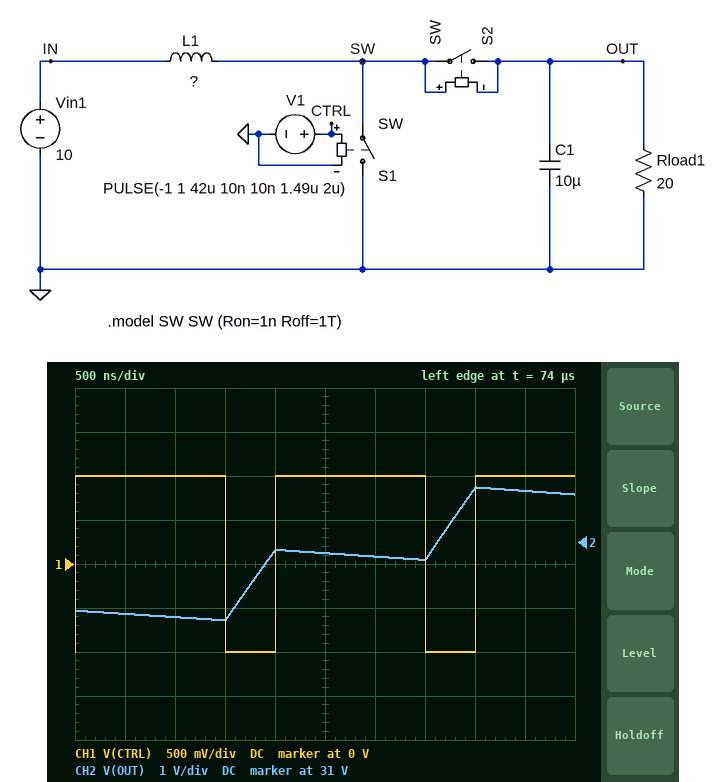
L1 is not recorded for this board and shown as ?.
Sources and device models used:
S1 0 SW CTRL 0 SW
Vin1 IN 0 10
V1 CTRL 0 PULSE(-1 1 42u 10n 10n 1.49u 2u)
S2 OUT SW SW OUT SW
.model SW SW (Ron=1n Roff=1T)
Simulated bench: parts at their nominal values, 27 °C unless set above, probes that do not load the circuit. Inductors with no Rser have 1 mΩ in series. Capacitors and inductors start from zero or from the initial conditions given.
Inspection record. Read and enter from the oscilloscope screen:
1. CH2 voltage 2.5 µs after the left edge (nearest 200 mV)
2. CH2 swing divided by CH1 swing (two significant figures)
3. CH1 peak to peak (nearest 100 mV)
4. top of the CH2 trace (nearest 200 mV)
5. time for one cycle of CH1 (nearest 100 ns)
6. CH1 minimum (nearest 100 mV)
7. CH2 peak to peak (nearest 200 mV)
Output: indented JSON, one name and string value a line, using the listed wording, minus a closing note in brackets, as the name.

{
  "CH2 voltage 2.5 µs after the left edge": "30.8 V",
  "CH2 swing divided by CH1 swing": "1.5",
  "CH1 peak to peak": "2.0 V",
  "top of the CH2 trace": "32.2 V",
  "time for one cycle of CH1": "2.0 µs",
  "CH1 minimum": "-1.0 V",
  "CH2 peak to peak": "3.0 V"
}
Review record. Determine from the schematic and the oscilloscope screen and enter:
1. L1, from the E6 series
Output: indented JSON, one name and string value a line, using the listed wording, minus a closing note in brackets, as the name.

{
  "L1, from the E6 series": "4.7 µH"
}
